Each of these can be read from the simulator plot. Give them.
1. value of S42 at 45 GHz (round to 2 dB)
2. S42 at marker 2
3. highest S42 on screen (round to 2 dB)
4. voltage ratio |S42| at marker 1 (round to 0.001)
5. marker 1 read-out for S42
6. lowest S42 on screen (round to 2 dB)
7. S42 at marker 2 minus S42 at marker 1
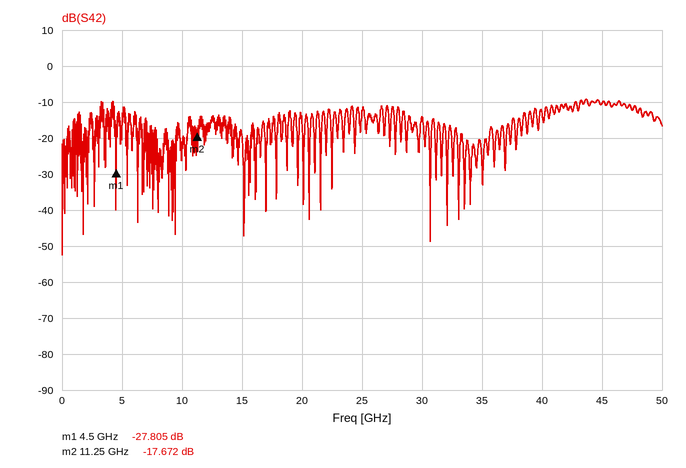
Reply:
-10 dB
-17.672 dB
-10 dB
0.041
-27.805 dB
-52 dB
10.133 dB
